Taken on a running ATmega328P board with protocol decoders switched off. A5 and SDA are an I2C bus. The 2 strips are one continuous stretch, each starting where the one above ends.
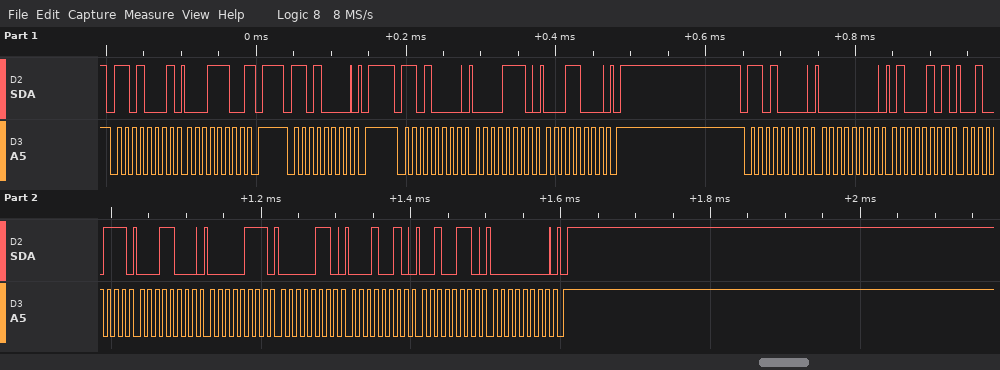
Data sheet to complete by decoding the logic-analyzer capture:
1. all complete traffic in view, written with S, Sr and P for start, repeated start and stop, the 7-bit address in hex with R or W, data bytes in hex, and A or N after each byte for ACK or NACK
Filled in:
S 68R A 1C N P S 68W A P S 68W A 0E A 18 A P S 68W A 00 A 45 A 27 A 18 A 07 A 06 A 12 A 26 A 00 A P
